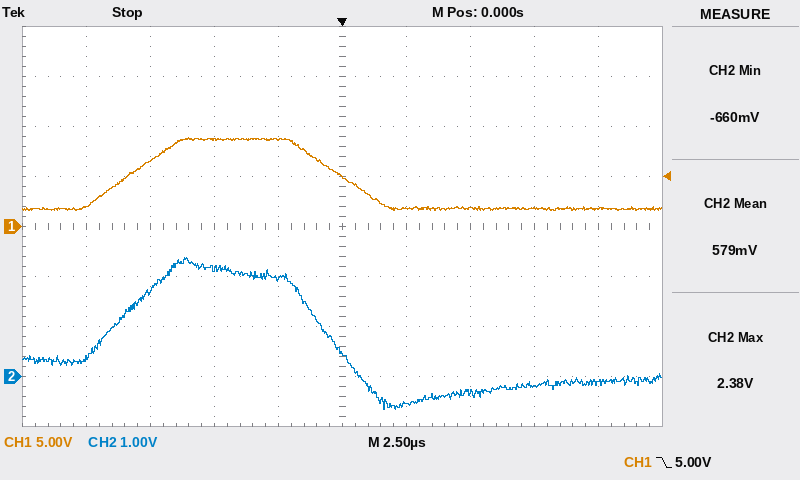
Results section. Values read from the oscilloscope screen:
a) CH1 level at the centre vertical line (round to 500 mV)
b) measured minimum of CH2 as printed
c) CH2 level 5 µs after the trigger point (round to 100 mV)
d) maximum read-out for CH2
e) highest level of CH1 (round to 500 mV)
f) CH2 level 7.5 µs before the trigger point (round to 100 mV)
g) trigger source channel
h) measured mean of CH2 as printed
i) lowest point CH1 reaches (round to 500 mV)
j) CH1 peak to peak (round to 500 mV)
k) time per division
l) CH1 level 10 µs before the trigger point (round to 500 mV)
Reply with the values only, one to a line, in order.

5.0 V
-660 mV
-300 mV
2.38 V
9.0 V
1.7 V
CH1
579 mV
1.5 V
7.5 V
2.5 µs
2.0 V
